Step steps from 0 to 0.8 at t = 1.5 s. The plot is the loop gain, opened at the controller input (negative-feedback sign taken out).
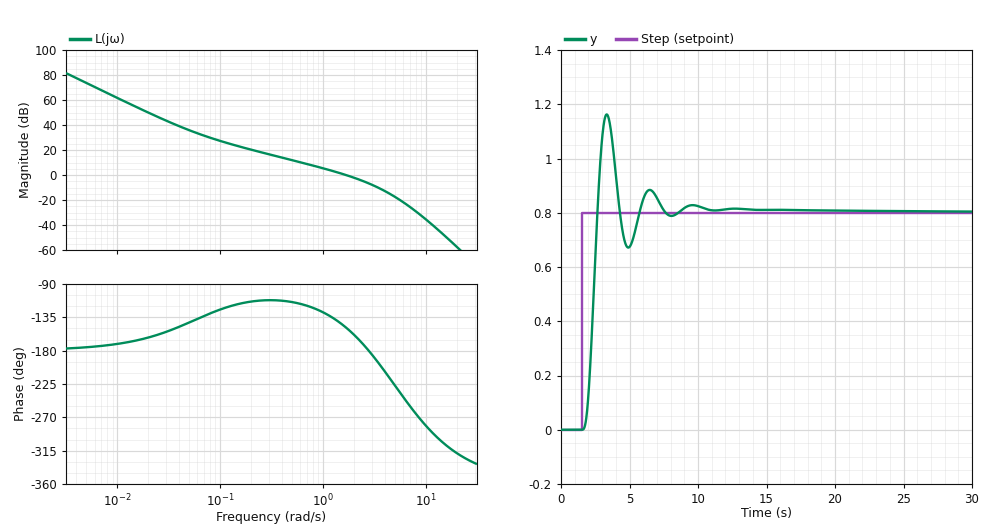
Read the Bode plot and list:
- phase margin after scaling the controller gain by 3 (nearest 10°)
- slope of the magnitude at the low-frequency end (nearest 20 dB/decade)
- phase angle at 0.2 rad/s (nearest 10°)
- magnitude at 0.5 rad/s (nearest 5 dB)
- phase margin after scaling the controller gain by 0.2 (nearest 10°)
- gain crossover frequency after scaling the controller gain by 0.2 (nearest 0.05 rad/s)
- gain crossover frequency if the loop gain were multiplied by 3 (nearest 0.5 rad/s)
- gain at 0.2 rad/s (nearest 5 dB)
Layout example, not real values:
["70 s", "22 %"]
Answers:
["-10°", "-40 dB/decade", "-110°", "10 dB", "70°", "0.40 rad/s", "3.5 rad/s", "20 dB"]
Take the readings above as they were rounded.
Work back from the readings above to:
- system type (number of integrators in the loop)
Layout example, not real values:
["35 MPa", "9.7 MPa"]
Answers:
["2"]
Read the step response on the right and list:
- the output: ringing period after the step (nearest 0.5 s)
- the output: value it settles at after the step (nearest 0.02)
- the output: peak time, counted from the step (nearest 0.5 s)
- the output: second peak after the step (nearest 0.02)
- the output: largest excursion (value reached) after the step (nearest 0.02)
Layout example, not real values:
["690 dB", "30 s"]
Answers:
["3.0 s", "0.80", "2.0 s", "0.88", "1.16"]
